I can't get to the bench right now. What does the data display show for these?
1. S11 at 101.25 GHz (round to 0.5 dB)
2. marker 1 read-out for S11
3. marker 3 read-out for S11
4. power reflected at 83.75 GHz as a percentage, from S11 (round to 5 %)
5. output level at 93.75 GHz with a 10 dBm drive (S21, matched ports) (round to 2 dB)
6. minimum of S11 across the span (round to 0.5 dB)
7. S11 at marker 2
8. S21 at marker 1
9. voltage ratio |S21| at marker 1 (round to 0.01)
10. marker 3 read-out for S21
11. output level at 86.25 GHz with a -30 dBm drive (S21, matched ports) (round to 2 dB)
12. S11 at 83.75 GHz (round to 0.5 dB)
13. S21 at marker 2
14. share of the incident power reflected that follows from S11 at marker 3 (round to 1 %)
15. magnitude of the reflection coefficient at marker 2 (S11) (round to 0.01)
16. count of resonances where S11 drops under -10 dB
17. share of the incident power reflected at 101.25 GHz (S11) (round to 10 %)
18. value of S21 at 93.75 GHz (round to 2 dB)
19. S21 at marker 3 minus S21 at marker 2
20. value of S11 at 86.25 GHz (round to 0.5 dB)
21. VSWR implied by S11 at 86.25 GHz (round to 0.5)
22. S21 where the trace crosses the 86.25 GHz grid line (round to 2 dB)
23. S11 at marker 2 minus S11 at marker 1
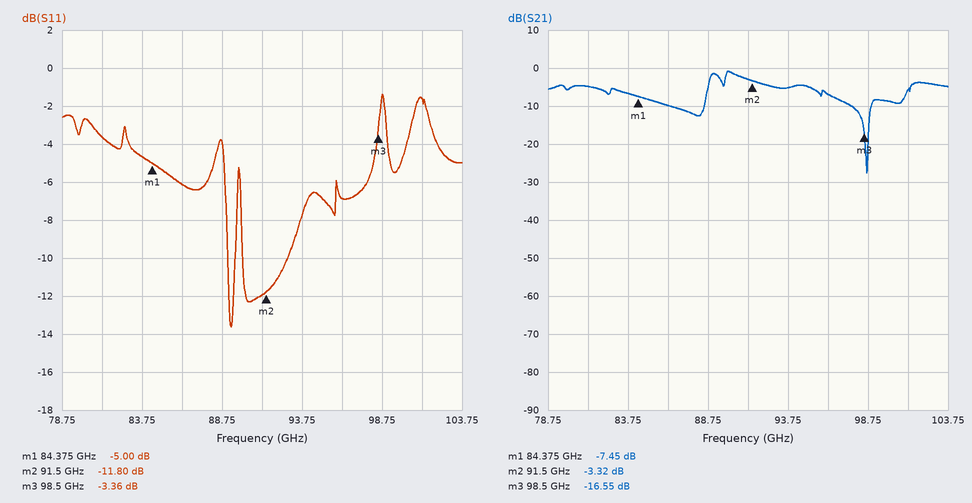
-1.5 dB
-5.00 dB
-3.36 dB
35 %
4 dBm
-13.5 dB
-11.80 dB
-7.45 dB
0.42
-16.55 dB
-40 dBm
-4.5 dB
-3.32 dB
46 %
0.26
2
70 %
-6 dB
-13.23 dB
-6.0 dB
3.0
-10 dB
-6.80 dB
